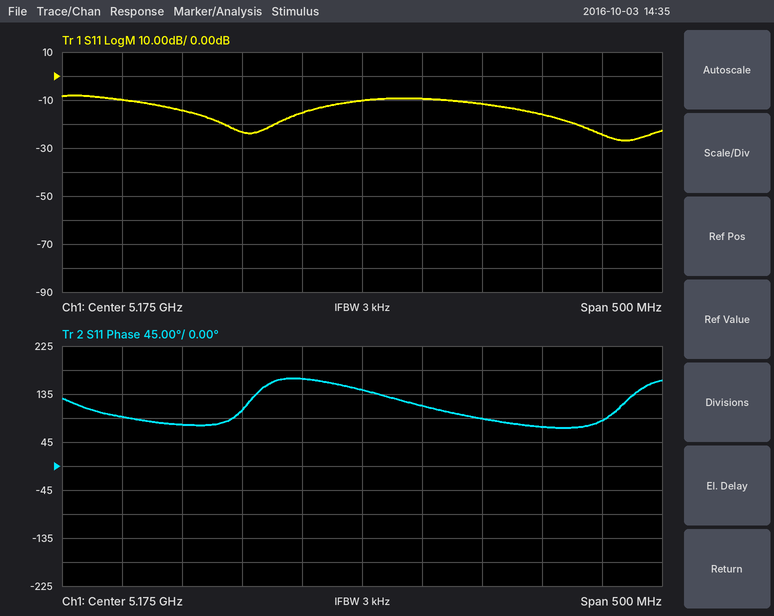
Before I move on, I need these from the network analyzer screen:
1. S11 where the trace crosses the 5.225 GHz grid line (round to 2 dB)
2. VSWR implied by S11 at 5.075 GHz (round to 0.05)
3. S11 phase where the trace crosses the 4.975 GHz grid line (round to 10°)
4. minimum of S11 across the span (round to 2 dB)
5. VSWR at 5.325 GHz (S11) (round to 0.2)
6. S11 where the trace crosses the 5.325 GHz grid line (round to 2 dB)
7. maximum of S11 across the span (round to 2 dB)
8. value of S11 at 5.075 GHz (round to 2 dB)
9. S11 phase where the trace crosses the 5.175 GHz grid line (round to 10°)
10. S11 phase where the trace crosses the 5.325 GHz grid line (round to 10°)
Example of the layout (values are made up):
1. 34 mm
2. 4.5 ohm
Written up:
1. -10 dB
2. 1.15
3. 90°
4. -26 dB
5. 1.4
6. -16 dB
7. -8 dB
8. -24 dB
9. 140°
10. 70°
